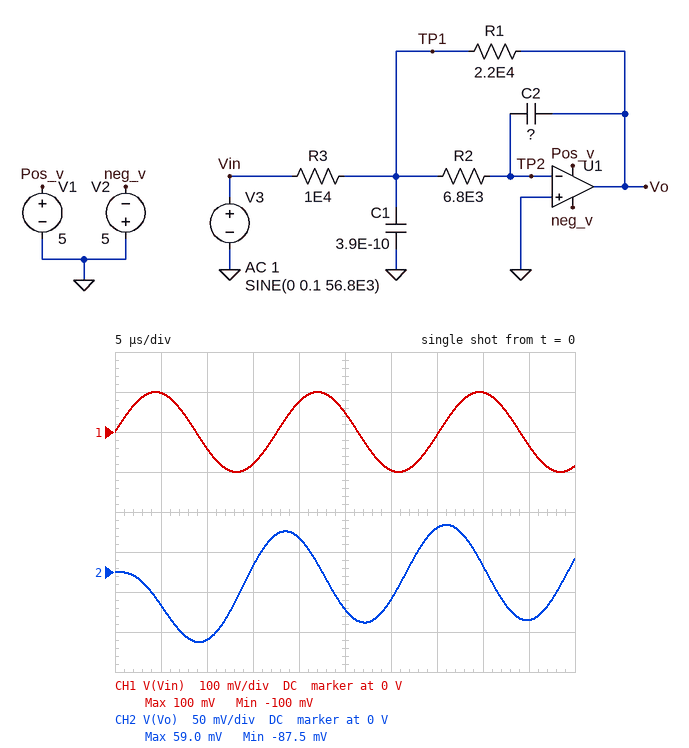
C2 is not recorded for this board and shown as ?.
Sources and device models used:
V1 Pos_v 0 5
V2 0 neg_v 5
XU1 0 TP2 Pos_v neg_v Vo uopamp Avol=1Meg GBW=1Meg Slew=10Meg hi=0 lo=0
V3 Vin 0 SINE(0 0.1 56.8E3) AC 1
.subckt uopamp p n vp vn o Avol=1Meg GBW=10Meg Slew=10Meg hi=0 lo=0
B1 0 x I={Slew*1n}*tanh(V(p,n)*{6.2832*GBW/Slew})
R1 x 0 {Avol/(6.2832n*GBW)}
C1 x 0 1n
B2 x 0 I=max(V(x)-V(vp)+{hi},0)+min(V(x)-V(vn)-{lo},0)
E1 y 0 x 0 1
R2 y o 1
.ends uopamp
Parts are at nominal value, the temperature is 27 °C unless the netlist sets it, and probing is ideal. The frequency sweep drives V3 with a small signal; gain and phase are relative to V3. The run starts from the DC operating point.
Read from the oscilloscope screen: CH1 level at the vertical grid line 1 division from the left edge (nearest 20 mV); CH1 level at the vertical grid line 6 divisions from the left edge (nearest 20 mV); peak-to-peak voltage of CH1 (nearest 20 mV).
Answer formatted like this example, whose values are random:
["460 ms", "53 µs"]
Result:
["100 mV", "-100 mV", "200 mV"]
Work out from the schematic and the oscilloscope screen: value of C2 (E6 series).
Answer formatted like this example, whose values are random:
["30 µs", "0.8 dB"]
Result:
["220 pF"]
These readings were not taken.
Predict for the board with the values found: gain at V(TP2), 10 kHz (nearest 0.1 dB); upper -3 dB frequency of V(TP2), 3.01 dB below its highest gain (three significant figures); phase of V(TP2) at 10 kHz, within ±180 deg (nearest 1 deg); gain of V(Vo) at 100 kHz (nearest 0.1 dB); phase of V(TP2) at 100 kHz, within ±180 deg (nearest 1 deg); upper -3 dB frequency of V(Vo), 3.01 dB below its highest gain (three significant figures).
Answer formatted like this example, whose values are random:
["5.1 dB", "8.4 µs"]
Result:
["-34.2 dB", "124 kHz", "56 deg", "-11.0 dB", "-42 deg", "18.5 kHz"]
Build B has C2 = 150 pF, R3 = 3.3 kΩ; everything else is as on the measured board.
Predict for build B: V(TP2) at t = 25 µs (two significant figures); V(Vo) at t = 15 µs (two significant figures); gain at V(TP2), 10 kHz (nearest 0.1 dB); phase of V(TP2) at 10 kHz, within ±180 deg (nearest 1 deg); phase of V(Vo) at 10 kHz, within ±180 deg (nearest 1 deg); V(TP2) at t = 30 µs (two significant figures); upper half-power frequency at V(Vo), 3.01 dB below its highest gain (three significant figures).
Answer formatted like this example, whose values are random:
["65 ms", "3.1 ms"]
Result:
["4.8 mV", "31 mV", "-25.3 dB", "51 deg", "141 deg", "-8.1 mV", "14.0 kHz"]
